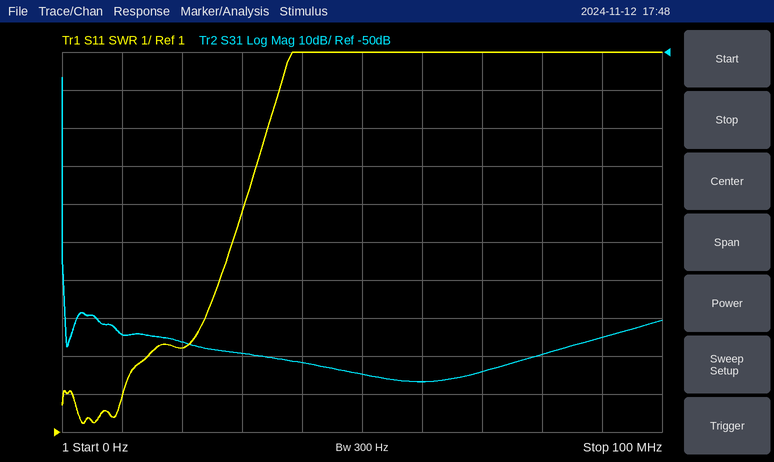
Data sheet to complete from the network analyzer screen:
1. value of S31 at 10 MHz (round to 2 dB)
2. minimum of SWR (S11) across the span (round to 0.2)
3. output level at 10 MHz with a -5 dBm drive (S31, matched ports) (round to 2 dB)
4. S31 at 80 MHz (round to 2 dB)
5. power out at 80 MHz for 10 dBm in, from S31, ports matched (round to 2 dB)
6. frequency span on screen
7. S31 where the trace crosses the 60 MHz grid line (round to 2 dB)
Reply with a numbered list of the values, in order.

1. -124 dB
2. 1.2
3. -130 dBm
4. -130 dB
5. -120 dBm
6. 100 MHz
7. -136 dB
